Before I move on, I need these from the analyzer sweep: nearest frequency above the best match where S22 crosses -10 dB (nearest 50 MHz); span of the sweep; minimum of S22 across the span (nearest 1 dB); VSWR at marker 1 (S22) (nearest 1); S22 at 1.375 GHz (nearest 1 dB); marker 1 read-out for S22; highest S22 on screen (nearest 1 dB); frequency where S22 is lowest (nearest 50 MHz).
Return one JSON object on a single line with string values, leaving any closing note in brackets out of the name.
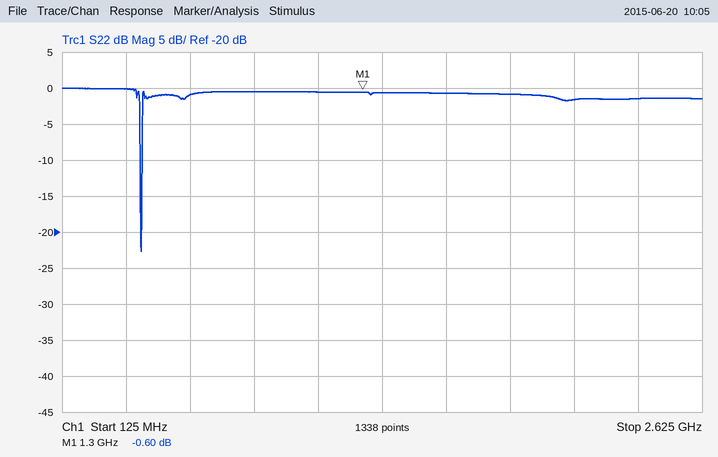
{"nearest frequency above the best match where S22 crosses -10 dB": "450 MHz", "span of the sweep": "2.5 GHz", "minimum of S22 across the span": "-23 dB", "VSWR at marker 1 (S22)": "29", "S22 at 1.375 GHz": "-1 dB", "marker 1 read-out for S22": "-0.60 dB", "highest S22 on screen": "0 dB", "frequency where S22 is lowest": "450 MHz"}
